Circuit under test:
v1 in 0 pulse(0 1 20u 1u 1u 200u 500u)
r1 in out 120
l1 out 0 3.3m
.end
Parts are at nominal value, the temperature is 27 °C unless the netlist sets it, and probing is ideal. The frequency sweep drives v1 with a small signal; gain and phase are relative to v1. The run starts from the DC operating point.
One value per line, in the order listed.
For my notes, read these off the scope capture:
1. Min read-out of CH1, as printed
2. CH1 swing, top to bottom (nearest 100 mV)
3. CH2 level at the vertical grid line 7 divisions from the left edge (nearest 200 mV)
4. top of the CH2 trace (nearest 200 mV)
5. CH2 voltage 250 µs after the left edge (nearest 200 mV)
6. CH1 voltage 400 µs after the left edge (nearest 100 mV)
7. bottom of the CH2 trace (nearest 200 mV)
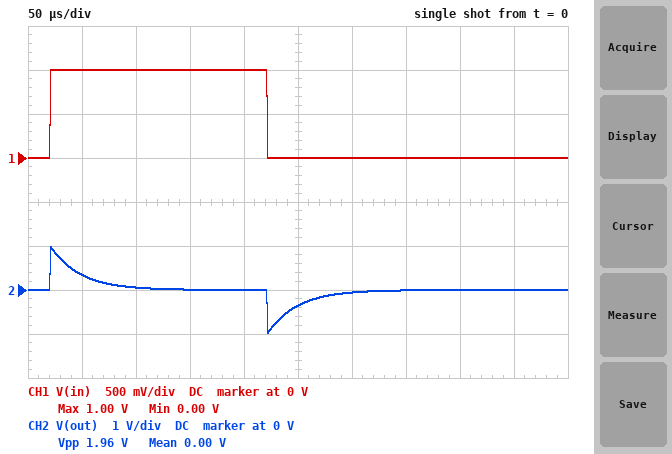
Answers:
0.00 V
1.0 V
0 V
1.0 V
-400 mV
0 V
-1.0 V
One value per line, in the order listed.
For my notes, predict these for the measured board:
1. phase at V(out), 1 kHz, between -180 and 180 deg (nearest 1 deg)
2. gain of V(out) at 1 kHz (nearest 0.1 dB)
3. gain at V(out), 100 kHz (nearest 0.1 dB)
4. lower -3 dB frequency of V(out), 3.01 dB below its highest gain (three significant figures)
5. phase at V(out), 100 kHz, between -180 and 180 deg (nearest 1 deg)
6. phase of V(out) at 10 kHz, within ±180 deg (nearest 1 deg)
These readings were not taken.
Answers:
80 deg
-15.4 dB
0 dB
5.79 kHz
3 deg
30 deg
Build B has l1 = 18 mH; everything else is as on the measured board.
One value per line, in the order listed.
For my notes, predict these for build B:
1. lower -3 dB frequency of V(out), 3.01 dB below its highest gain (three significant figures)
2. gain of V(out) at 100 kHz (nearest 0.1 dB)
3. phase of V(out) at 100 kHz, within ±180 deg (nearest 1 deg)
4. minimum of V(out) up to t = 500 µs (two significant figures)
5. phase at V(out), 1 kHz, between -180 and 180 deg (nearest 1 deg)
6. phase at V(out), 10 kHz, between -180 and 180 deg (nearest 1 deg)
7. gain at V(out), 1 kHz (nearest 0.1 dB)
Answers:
1.06 kHz
0 dB
1 deg
-740 mV
47 deg
6 deg
-3.3 dB
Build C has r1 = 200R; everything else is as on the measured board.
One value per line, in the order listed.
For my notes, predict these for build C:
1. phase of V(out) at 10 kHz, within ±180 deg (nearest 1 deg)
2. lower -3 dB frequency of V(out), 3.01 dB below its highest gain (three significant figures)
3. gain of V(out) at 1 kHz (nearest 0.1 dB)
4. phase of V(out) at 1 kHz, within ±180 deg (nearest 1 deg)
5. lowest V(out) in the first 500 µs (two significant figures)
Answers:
44 deg
9.65 kHz
-19.7 dB
84 deg
-970 mV
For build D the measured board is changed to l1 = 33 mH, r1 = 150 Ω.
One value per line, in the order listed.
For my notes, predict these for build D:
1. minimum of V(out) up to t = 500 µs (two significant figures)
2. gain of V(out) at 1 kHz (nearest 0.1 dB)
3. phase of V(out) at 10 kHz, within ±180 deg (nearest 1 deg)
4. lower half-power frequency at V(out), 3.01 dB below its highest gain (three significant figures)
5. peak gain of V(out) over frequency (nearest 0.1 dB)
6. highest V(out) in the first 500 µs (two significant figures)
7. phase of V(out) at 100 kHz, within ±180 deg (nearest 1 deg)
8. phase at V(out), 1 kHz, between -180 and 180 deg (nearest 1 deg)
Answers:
-600 mV
-1.8 dB
4 deg
723 Hz
0 dB
1.0 V
0 deg
36 deg
